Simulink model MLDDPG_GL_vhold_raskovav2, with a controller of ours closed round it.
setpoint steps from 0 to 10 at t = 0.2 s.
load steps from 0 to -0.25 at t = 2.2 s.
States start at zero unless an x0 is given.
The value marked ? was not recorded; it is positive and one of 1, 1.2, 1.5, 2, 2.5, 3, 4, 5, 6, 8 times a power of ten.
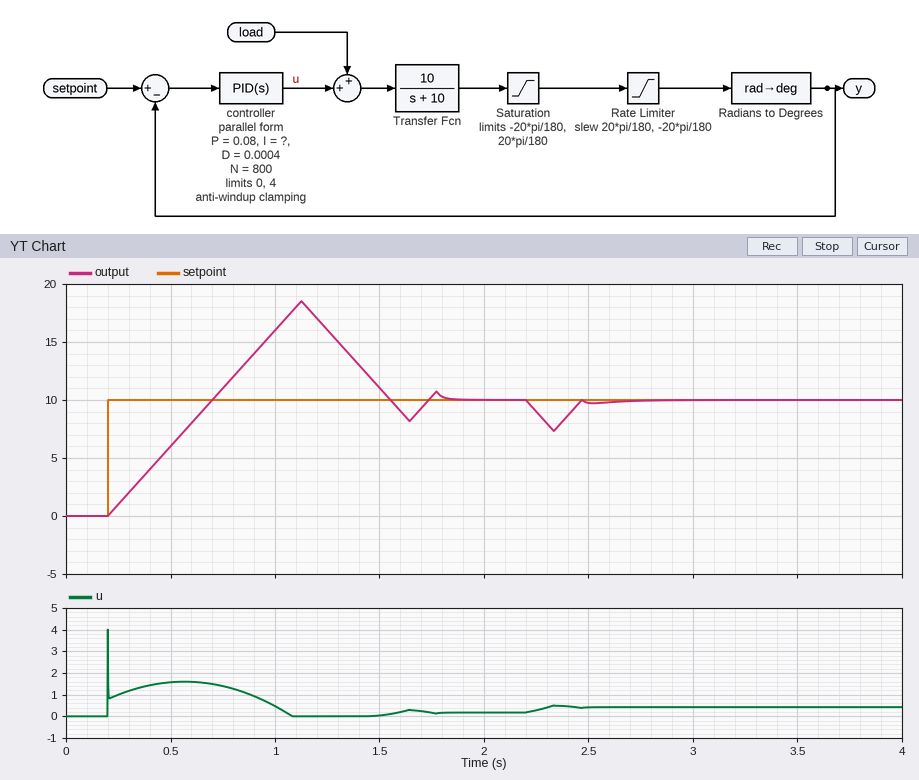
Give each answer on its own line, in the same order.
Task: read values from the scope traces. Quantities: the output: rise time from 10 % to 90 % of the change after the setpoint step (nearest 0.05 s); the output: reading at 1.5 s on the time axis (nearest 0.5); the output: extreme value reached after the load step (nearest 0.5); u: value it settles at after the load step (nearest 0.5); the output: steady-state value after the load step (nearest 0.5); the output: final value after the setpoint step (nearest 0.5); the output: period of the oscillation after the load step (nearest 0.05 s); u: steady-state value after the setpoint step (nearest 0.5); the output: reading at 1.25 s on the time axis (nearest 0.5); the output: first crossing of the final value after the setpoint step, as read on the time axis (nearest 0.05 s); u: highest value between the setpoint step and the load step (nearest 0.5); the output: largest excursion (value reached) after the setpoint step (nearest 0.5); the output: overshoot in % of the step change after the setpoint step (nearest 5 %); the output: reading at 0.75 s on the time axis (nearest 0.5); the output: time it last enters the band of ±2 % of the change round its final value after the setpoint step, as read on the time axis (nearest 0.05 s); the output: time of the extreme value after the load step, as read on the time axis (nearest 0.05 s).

0.40 s
11.0
7.5
0.5
10.0
10.0
0.20 s
0.0
16.0
0.70 s
4.0
18.5
85 %
11.0
1.80 s
2.35 s
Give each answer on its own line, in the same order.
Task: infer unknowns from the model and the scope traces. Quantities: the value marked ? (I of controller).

0.6
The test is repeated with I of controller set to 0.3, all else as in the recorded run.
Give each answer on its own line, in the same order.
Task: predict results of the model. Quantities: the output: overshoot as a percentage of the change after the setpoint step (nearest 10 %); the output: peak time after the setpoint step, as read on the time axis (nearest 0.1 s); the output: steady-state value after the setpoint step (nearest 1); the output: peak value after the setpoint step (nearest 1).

60 %
1.0 s
10
16
